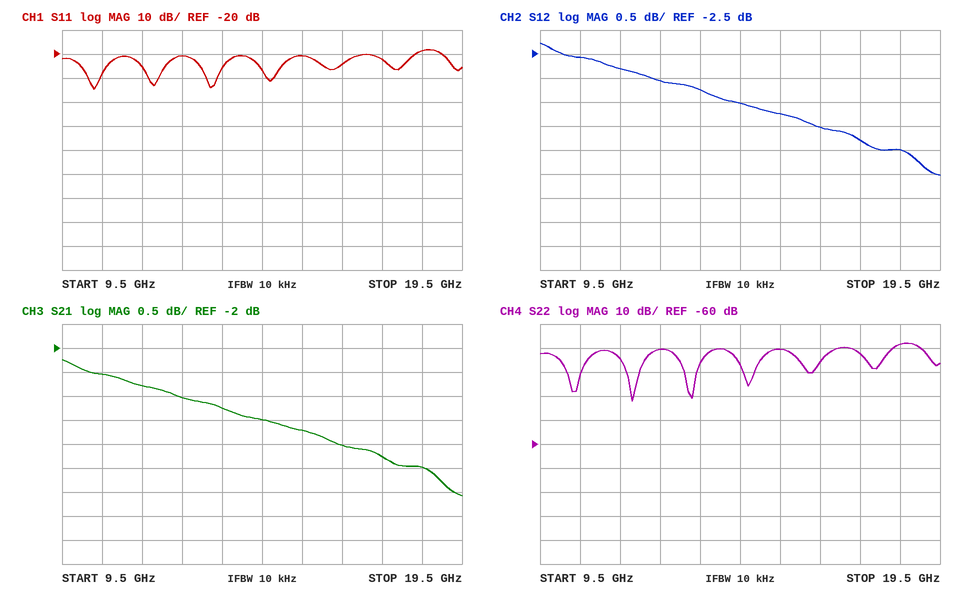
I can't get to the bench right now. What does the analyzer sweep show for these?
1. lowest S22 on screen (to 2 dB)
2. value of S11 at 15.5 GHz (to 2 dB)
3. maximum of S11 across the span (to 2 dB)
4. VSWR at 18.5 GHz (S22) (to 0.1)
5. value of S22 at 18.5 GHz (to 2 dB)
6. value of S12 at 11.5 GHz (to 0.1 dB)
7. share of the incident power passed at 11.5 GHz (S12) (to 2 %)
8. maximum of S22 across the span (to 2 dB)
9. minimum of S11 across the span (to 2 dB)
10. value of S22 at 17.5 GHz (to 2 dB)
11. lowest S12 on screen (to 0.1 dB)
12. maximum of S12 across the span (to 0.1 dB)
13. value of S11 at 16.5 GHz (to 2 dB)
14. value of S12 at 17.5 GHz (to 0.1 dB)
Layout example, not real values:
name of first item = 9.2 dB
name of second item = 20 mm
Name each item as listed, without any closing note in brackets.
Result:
lowest S22 on screen = -42 dB
value of S11 at 15.5 GHz = -20 dB
maximum of S11 across the span = -18 dB
VSWR at 18.5 GHz (S22) = 1.3
value of S22 at 18.5 GHz = -18 dB
value of S12 at 11.5 GHz = -2.8 dB
share of the incident power passed at 11.5 GHz (S12) = 52 %
maximum of S22 across the span = -18 dB
minimum of S11 across the span = -34 dB
value of S22 at 17.5 GHz = -22 dB
lowest S12 on screen = -5.0 dB
maximum of S12 across the span = -2.3 dB
value of S11 at 16.5 GHz = -24 dB
value of S12 at 17.5 GHz = -4.3 dB
